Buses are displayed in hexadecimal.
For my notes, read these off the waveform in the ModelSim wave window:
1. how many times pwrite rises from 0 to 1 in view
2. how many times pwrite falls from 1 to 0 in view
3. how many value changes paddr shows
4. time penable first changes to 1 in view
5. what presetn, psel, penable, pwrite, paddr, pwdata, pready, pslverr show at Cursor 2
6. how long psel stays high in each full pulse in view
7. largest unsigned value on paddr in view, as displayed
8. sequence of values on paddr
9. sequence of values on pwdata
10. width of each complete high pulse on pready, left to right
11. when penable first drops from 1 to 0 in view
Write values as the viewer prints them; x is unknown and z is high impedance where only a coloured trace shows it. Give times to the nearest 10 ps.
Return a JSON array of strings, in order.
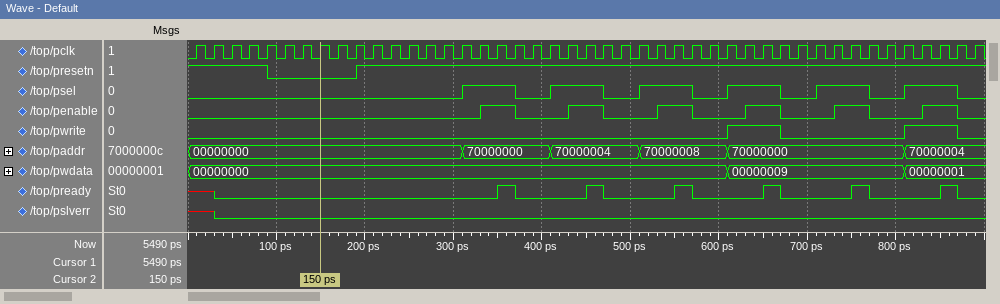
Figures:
["2", "2", "5", "330 ps", "presetn=0, psel=0, penable=0, pwrite=0, paddr=00000000, pwdata=00000000, pready=0, pslverr=0", "60 ps, 60 ps, 60 ps, 60 ps, 60 ps, 60 ps", "70000008", "00000000, 70000000, 70000004, 70000008, 70000000, 70000004", "00000000, 00000009, 00000001", "20 ps, 20 ps, 20 ps, 20 ps, 20 ps, 20 ps", "370 ps"]
